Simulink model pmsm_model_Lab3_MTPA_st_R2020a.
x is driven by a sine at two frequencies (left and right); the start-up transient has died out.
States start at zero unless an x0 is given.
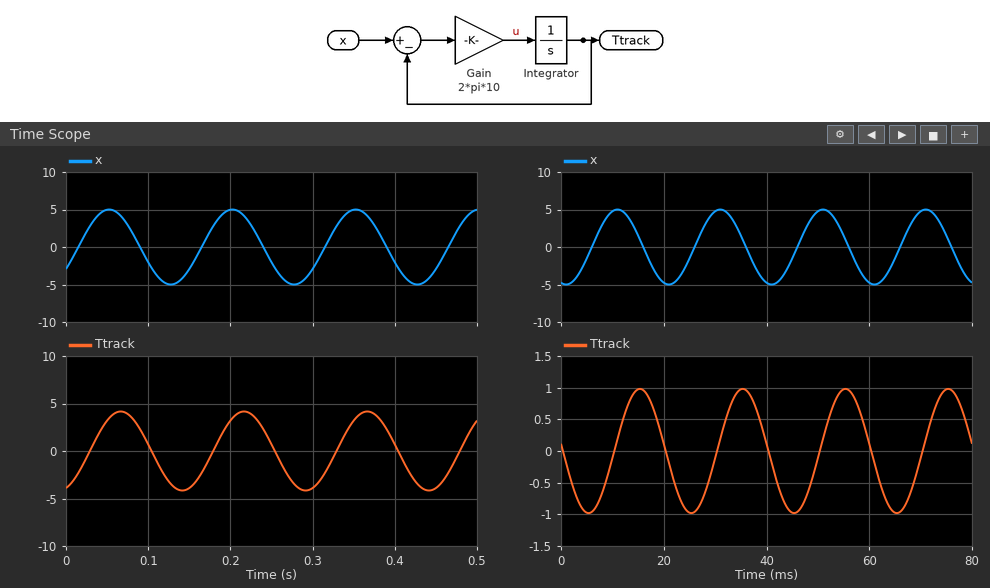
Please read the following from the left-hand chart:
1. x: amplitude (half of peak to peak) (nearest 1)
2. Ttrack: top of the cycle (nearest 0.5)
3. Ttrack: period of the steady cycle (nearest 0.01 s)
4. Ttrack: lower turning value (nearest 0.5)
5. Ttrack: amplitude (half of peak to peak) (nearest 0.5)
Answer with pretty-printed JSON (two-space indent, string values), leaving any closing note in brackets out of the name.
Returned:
{
  "x: amplitude (half of peak to peak)": "5",
  "Ttrack: top of the cycle": "4.0",
  "Ttrack: period of the steady cycle": "0.15 s",
  "Ttrack: lower turning value": "-4.0",
  "Ttrack: amplitude (half of peak to peak)": "4.0"
}
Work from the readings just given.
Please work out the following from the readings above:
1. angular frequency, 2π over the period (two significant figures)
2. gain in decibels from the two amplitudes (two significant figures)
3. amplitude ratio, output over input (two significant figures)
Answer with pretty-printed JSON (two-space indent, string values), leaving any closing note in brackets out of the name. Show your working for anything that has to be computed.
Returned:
{
  "angular frequency, 2π over the period": "2π / 0.15 = 42 rad/s",
  "gain in decibels from the two amplitudes": "20 log10(4 / 5) = -1.9 dB",
  "amplitude ratio, output over input": "4 / 5 = 0.80"
}
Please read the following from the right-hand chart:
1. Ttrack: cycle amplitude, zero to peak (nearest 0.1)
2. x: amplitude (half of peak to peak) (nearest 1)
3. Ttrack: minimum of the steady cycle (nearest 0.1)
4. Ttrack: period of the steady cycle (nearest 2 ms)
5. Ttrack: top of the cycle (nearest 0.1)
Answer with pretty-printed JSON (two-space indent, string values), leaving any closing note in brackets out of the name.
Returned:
{
  "Ttrack: cycle amplitude, zero to peak": "1.0",
  "x: amplitude (half of peak to peak)": "5",
  "Ttrack: minimum of the steady cycle": "-1.0",
  "Ttrack: period of the steady cycle": "20 ms",
  "Ttrack: top of the cycle": "1.0"
}
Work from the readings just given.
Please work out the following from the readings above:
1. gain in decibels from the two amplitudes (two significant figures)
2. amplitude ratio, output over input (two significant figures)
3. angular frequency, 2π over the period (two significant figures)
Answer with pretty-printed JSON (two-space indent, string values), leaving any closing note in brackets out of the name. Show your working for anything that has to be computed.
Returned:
{
  "gain in decibels from the two amplitudes": "20 log10(1 / 5) = -14 dB",
  "amplitude ratio, output over input": "1 / 5 = 0.20",
  "angular frequency, 2π over the period": "2π / 20 = 0.31 rad/ms"
}
